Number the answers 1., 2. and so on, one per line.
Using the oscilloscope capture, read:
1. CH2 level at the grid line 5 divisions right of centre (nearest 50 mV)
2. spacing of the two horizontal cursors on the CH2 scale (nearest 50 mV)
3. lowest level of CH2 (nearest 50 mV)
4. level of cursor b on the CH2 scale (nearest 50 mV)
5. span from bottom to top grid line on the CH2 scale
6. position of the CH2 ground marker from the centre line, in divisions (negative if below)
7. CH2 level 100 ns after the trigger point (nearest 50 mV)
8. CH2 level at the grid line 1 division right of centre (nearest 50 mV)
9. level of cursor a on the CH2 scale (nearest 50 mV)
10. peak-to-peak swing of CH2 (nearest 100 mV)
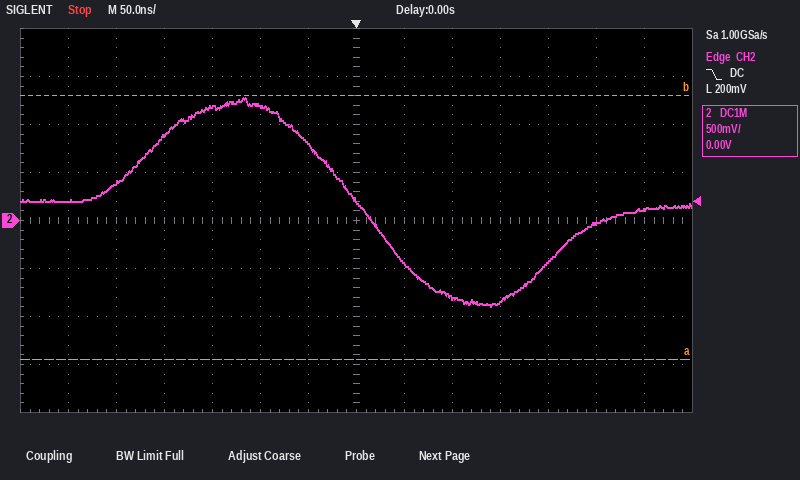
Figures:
1. -50 mV
2. 2.75 V
3. -900 mV
4. 1.30 V
5. 4 V
6. 0.0 div
7. -800 mV
8. -450 mV
9. -1.45 V
10. 2.20 V
